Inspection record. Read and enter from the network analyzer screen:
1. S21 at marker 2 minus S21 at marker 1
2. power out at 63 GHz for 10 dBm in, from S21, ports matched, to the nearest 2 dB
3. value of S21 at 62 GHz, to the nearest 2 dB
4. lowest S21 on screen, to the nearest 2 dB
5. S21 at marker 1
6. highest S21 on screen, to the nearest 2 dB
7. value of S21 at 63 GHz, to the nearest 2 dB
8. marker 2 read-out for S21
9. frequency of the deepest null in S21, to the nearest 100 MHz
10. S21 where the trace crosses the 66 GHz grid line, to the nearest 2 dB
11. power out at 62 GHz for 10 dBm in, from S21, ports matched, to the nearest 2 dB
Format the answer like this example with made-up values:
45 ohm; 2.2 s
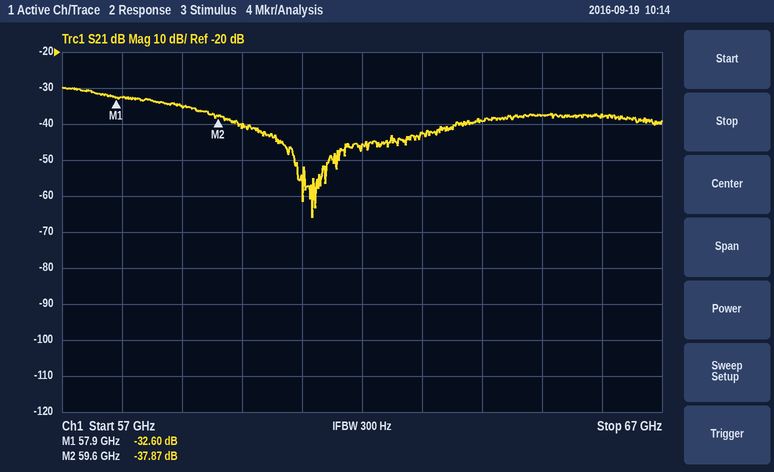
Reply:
-5.27 dB; -32 dBm; -46 dB; -66 dB; -32.60 dB; -30 dB; -42 dB; -37.87 dB; 61.2 GHz; -38 dB; -36 dBm
